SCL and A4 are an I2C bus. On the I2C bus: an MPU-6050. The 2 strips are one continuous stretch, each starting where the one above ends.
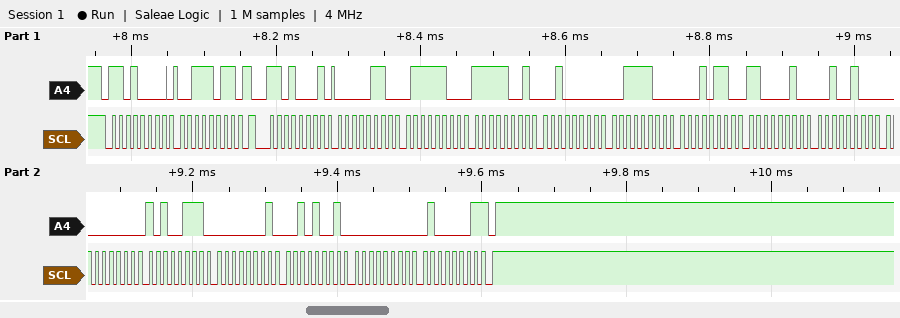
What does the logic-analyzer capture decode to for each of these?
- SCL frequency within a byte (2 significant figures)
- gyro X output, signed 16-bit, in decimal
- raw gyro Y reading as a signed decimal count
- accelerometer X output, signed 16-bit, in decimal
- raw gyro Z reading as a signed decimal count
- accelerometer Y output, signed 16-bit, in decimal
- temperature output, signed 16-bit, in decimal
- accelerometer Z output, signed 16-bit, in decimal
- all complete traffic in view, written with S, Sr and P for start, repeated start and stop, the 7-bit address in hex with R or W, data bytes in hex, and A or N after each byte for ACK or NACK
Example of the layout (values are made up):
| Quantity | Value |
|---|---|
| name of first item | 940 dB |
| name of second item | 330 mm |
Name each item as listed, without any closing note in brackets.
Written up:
| Quantity | Value |
|---|---|
| SCL frequency within a byte | 100 kHz |
| gyro X output, signed 16-bit, in decimal | 167 |
| raw gyro Y reading as a signed decimal count | 297 |
| accelerometer X output, signed 16-bit, in decimal | 1660 |
| raw gyro Z reading as a signed decimal count | 65 |
| accelerometer Y output, signed 16-bit, in decimal | -1760 |
| temperature output, signed 16-bit, in decimal | -15836 |
| accelerometer Z output, signed 16-bit, in decimal | 15382 |
| all complete traffic in view, written with S, Sr and P for start, repeated start and stop, the 7-bit address in hex with R or W, data bytes in hex, and A or N after each byte for ACK or NACK | S 68W A 3B A Sr 68R A 06 A 7C A F9 A 20 A 3C A 16 A C2 A 24 A 00 A A7 A 01 A 29 A 00 A 41 N P |
